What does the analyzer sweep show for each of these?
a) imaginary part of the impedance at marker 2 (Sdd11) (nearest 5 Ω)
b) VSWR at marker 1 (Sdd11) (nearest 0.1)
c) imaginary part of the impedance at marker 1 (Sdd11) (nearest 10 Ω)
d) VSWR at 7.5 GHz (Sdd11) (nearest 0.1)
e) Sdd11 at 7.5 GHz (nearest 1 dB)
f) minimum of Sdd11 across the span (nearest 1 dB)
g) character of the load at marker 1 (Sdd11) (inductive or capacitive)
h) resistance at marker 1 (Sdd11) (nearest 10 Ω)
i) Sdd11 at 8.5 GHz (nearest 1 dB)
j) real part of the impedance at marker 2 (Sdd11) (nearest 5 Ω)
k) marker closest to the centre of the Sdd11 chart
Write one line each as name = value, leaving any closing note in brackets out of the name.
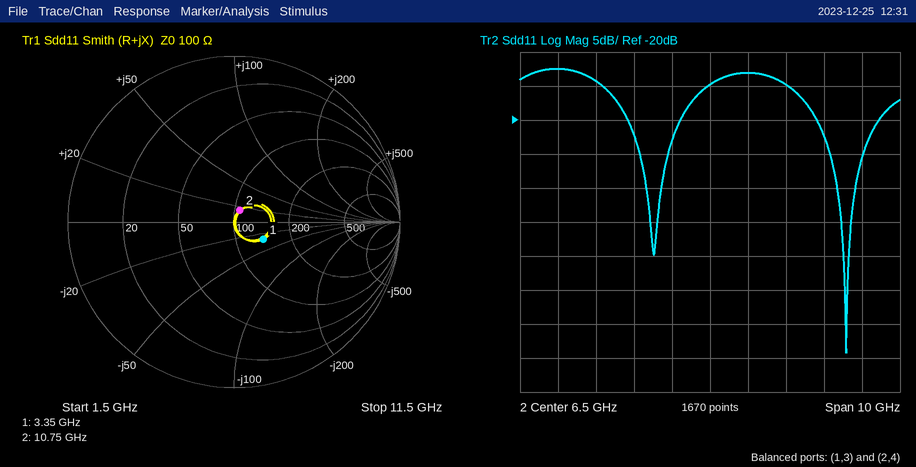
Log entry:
imaginary part of the impedance at marker 2 (Sdd11) = +15 Ω
VSWR at marker 1 (Sdd11) = 1.5
imaginary part of the impedance at marker 1 (Sdd11) = -30 Ω
VSWR at 7.5 GHz (Sdd11) = 1.6
Sdd11 at 7.5 GHz = -13 dB
minimum of Sdd11 across the span = -54 dB
character of the load at marker 1 (Sdd11) = capacitive
resistance at marker 1 (Sdd11) = 140 Ω
Sdd11 at 8.5 GHz = -15 dB
real part of the impedance at marker 2 (Sdd11) = 105 Ω
marker closest to the centre of the Sdd11 chart = marker 2
